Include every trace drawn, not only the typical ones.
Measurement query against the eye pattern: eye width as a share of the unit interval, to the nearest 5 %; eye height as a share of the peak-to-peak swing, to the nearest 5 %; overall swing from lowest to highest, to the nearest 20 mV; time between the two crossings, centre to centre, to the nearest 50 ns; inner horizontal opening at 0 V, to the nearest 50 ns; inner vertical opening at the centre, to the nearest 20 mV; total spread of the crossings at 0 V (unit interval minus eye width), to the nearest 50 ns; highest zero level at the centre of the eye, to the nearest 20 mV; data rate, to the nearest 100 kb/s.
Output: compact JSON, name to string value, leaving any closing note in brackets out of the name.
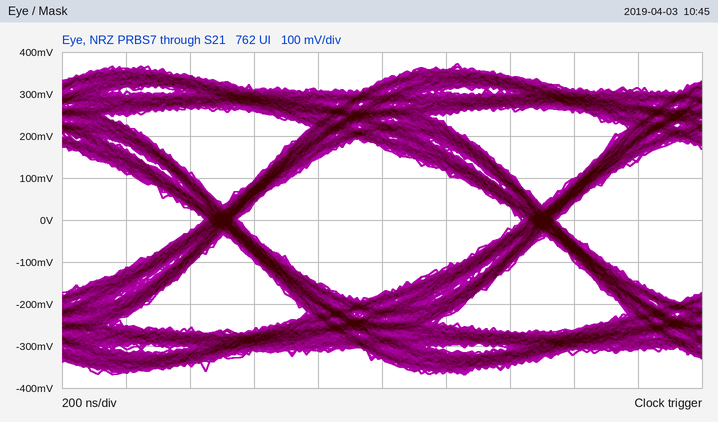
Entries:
{"eye width as a share of the unit interval, to the nearest 5 %": "90 %", "eye height as a share of the peak-to-peak swing, to the nearest 5 %": "45 %", "overall swing from lowest to highest, to the nearest 20 mV": "740 mV", "time between the two crossings, centre to centre, to the nearest 50 ns": "1.00 µs", "inner horizontal opening at 0 V, to the nearest 50 ns": "900 ns", "inner vertical opening at the centre, to the nearest 20 mV": "340 mV", "total spread of the crossings at 0 V (unit interval minus eye width), to the nearest 50 ns": "100 ns", "highest zero level at the centre of the eye, to the nearest 20 mV": "-180 mV", "data rate, to the nearest 100 kb/s": "1.0 Mb/s"}
